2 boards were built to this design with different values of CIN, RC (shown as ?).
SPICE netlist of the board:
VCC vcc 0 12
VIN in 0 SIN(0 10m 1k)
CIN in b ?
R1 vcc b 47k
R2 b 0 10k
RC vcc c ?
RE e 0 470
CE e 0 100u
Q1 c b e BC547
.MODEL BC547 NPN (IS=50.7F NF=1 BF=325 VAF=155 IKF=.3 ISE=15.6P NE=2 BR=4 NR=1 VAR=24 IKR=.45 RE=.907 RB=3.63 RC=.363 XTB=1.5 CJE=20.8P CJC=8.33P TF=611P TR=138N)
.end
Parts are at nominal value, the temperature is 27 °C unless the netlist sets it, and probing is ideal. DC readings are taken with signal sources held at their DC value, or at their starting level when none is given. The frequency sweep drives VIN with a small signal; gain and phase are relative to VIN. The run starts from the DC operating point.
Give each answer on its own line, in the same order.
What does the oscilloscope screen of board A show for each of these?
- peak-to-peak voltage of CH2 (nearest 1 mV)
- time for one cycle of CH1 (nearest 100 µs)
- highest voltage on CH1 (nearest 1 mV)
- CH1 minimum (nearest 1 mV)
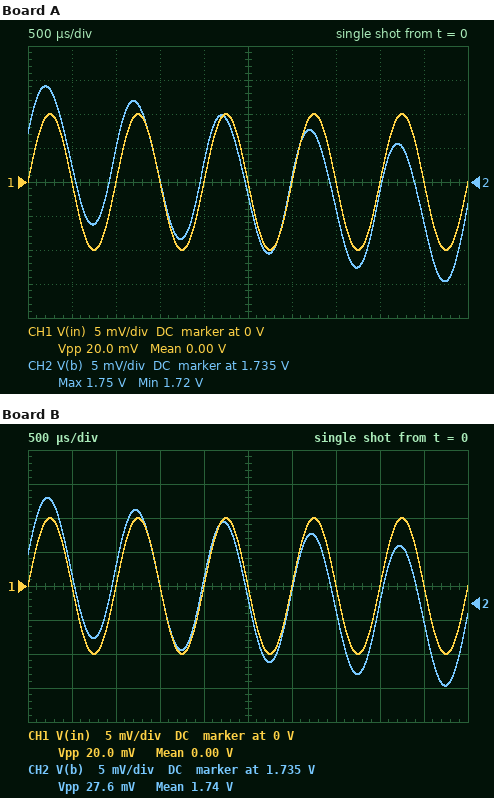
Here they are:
29 mV
1.0 ms
10 mV
-10 mV
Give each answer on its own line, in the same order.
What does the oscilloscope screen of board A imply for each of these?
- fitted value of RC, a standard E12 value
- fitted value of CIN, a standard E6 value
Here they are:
4.7 kΩ
6.8 µF
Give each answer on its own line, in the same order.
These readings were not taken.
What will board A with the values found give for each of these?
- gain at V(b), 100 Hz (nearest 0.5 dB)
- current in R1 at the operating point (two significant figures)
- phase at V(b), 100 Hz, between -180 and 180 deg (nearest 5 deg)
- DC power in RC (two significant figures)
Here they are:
-12.5 dB
220 µA
60 deg
25 mW
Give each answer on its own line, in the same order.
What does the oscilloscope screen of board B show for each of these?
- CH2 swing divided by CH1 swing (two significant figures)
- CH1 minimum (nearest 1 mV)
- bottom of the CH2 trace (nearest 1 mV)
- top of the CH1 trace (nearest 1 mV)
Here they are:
1.4
-10 mV
1.723 V
10 mV
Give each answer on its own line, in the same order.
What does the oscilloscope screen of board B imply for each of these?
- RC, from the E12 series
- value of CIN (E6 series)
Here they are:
4.7 kΩ
15 µF
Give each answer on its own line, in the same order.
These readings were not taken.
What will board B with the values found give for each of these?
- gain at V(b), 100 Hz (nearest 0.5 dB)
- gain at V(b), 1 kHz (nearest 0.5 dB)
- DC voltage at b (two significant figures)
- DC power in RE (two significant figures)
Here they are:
-7.0 dB
0 dB
1.7 V
2.6 mW
